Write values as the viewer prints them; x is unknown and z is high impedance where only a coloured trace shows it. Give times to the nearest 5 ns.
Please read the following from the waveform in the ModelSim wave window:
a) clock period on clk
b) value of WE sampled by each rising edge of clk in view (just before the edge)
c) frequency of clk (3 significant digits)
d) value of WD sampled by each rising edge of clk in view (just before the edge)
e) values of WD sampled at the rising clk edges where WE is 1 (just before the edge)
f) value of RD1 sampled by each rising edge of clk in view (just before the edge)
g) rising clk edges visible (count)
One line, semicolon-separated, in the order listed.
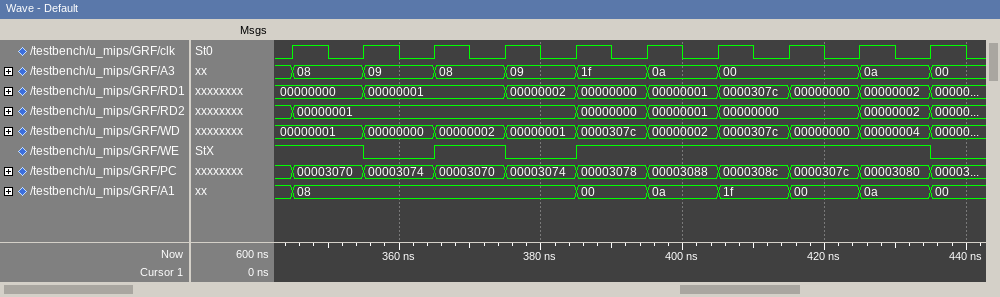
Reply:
10 ns; 1 1 0 1 0 1 1 1 1 1; 100 MHz; 00000001, 00000001, 00000000, 00000002, 00000001, 0000307c, 00000002, 0000307c, 00000000, 00000004; 00000001, 00000001, 00000002, 0000307c, 00000002, 0000307c, 00000000, 00000004; 00000000, 00000000, 00000001, 00000001, 00000002, 00000000, 00000001, 0000307c, 00000000, 00000002; 10
